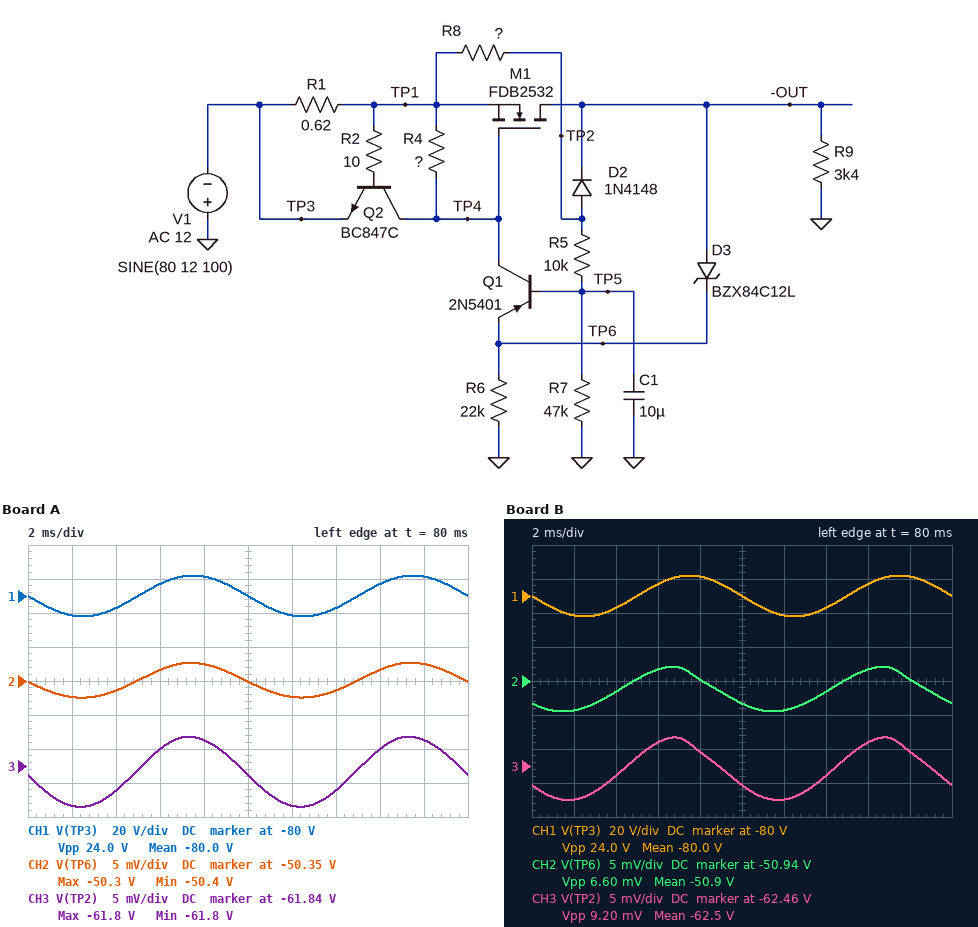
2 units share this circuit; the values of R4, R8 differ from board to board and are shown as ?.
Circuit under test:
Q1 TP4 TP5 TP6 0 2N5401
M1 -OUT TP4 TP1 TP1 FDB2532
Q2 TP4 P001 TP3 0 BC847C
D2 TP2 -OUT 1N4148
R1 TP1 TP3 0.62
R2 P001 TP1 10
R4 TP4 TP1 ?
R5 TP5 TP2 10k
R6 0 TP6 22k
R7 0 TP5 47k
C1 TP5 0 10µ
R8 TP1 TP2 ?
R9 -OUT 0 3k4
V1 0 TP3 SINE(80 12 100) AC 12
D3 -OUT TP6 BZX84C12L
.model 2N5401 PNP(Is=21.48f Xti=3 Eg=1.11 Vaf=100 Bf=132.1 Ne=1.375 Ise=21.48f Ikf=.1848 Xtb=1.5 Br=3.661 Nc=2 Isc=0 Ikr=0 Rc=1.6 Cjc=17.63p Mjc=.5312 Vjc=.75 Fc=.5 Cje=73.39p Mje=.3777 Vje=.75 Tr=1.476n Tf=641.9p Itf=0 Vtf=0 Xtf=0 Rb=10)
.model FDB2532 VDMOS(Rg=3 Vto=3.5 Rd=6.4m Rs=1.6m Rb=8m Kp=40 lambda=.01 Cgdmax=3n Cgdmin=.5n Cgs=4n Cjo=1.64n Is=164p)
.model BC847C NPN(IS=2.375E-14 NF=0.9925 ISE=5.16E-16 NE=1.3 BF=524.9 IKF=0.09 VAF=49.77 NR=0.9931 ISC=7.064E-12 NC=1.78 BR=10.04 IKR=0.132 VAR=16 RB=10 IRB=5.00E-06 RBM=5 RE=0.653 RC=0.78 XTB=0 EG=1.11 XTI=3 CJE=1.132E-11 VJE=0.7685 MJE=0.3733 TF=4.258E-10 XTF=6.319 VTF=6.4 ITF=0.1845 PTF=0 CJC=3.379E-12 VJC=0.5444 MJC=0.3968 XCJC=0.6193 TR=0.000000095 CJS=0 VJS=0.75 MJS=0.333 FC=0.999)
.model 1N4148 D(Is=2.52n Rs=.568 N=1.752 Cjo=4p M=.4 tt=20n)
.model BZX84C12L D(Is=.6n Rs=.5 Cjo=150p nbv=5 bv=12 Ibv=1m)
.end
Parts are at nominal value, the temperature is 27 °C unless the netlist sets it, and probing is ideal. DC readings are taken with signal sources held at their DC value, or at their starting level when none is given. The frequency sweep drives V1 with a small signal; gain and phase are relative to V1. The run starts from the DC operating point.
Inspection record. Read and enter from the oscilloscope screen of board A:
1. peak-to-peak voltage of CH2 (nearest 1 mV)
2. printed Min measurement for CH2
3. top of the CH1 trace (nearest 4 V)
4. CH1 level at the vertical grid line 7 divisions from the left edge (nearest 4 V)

5 mV
-50.4 V
-68 V
-88 V
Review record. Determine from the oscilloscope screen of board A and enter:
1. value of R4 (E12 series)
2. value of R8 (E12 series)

6.8 kΩ
220 kΩ
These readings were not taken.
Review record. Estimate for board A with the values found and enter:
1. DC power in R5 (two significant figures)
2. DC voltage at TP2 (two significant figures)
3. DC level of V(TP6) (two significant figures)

12 mW
-62 V
-50 V
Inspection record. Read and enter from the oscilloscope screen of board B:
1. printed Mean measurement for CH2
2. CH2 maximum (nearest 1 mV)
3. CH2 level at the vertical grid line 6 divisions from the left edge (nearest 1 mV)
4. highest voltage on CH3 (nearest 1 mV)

-50.9 V
-50.938 V
-50.944 V
-62.456 V
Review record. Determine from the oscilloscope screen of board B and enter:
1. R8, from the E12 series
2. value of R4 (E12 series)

390 kΩ
56 kΩ
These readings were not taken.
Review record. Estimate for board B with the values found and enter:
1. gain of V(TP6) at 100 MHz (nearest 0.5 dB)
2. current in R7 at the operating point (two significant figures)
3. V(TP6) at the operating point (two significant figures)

-9.5 dB
1.1 mA
-51 V
